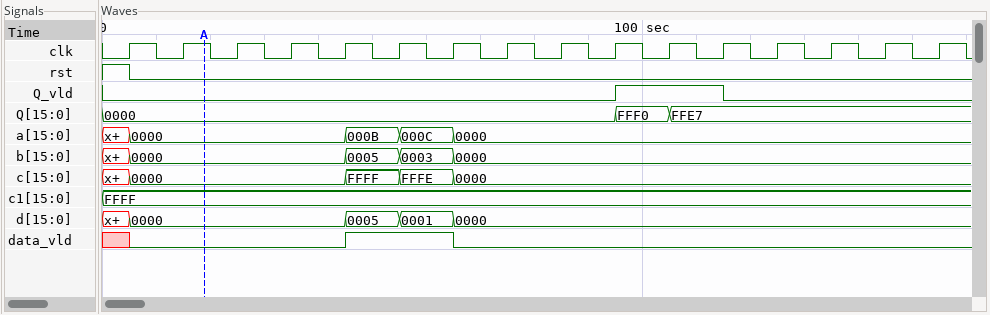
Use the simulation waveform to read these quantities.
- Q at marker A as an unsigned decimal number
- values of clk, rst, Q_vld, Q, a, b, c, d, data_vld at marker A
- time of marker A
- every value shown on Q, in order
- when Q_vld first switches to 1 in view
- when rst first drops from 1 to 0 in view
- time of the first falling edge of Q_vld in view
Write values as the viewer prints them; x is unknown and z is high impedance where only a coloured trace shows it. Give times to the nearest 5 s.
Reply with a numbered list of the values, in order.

1. 0
2. clk=1, rst=0, Q_vld=0, Q=0000, a=0000, b=0000, c=0000, d=0000, data_vld=0
3. 20 s
4. 0000, FFF0, FFE7
5. 95 s
6. 5 s
7. 115 s
